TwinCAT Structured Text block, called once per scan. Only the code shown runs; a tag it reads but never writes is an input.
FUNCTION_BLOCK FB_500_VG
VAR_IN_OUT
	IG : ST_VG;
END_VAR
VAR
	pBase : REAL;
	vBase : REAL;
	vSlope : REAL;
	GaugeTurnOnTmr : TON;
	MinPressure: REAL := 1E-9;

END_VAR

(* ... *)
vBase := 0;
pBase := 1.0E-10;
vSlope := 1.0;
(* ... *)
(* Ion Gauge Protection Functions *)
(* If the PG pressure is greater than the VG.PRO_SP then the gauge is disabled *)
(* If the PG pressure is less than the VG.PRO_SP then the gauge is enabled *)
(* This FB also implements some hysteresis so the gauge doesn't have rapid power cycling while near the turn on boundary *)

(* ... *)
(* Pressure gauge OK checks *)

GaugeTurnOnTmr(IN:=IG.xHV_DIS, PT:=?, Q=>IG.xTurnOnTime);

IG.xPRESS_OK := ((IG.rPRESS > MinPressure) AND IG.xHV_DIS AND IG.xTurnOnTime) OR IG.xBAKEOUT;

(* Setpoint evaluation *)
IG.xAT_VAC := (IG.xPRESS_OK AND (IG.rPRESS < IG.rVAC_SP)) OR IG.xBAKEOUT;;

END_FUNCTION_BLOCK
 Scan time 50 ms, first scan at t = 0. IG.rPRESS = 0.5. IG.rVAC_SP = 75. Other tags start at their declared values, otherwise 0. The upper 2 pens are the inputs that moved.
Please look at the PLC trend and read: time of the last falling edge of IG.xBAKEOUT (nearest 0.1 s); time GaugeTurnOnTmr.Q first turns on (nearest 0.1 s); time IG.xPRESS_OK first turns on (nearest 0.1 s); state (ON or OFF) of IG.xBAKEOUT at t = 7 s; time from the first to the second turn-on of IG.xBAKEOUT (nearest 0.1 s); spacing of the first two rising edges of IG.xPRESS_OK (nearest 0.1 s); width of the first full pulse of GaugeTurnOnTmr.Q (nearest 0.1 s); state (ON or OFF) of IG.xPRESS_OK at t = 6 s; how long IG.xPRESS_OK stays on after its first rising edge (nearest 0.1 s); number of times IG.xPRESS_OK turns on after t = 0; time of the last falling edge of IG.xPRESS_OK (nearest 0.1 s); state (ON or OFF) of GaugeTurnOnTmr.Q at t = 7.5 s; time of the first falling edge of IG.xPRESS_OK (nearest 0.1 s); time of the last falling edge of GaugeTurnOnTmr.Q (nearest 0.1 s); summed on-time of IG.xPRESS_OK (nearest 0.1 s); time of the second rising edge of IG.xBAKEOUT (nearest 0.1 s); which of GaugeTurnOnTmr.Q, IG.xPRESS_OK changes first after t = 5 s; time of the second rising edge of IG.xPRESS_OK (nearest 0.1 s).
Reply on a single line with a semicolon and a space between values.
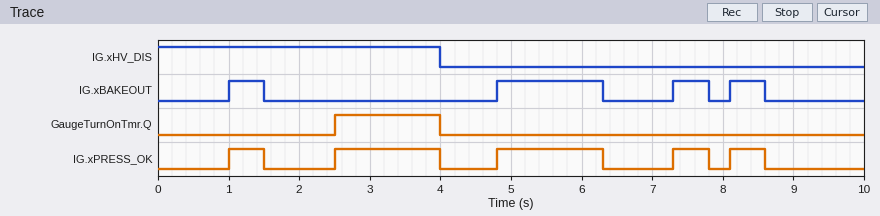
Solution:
8.6 s; 2.5 s; 1.0 s; OFF; 3.8 s; 1.5 s; 1.5 s; ON; 0.5 s; 5; 8.6 s; OFF; 1.5 s; 4.0 s; 4.5 s; 4.8 s; IG.xPRESS_OK; 2.5 s
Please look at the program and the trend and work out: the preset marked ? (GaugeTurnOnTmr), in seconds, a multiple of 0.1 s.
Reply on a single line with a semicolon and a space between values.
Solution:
2.5 s
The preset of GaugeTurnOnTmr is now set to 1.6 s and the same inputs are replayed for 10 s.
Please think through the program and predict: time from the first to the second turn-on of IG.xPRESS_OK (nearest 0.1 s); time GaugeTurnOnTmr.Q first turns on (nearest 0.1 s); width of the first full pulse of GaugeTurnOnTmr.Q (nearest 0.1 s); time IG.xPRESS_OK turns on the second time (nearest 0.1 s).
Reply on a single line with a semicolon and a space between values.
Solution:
0.6 s; 1.6 s; 2.4 s; 1.6 s
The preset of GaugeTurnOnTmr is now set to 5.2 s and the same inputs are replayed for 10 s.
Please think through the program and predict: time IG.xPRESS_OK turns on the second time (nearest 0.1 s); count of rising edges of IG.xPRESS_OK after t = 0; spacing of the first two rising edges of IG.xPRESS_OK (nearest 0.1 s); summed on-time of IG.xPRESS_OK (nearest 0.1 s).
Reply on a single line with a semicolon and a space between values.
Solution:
4.8 s; 4; 3.8 s; 3.0 s
